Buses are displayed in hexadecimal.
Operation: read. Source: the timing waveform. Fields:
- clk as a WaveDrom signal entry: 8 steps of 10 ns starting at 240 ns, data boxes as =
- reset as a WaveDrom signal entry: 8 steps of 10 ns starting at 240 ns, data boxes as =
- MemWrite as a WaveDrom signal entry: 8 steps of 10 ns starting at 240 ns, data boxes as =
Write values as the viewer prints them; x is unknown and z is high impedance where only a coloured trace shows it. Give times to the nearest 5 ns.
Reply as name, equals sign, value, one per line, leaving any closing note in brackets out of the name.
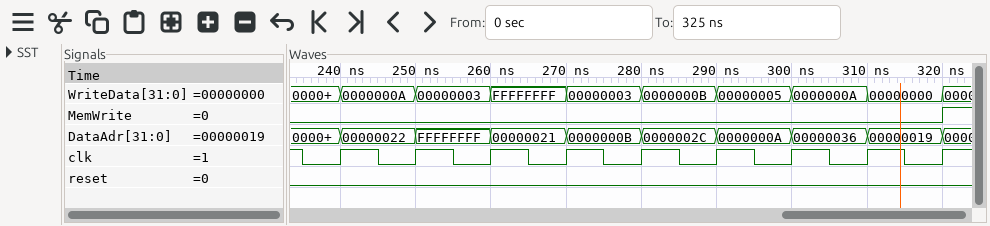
clk as a WaveDrom signal entry: 8 steps of 10 ns starting at 240 ns, data boxes as = = {name: 'clk', wave: 'p.......'}
reset as a WaveDrom signal entry: 8 steps of 10 ns starting at 240 ns, data boxes as = = {name: 'reset', wave: '0.......'}
MemWrite as a WaveDrom signal entry: 8 steps of 10 ns starting at 240 ns, data boxes as = = {name: 'MemWrite', wave: '0.......'}
